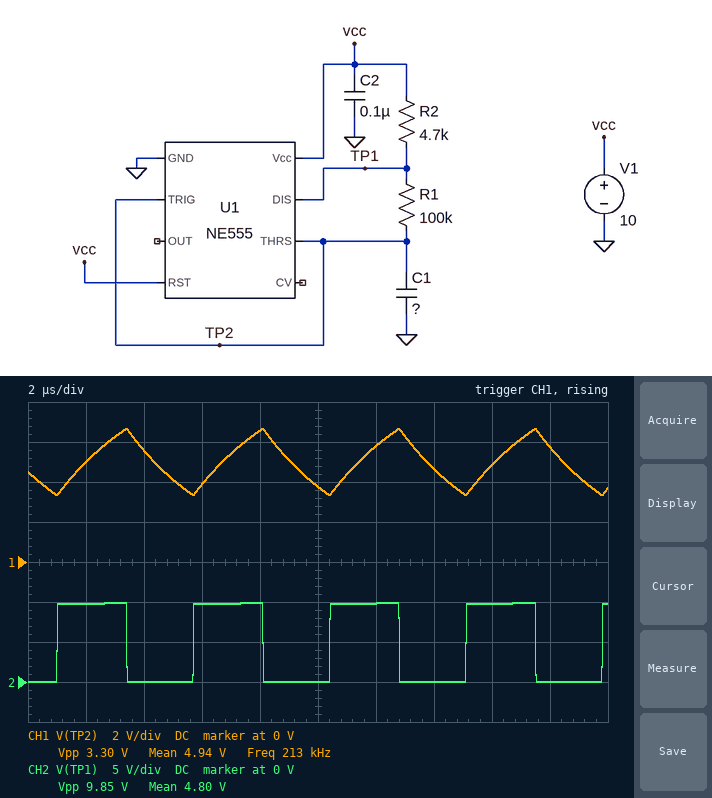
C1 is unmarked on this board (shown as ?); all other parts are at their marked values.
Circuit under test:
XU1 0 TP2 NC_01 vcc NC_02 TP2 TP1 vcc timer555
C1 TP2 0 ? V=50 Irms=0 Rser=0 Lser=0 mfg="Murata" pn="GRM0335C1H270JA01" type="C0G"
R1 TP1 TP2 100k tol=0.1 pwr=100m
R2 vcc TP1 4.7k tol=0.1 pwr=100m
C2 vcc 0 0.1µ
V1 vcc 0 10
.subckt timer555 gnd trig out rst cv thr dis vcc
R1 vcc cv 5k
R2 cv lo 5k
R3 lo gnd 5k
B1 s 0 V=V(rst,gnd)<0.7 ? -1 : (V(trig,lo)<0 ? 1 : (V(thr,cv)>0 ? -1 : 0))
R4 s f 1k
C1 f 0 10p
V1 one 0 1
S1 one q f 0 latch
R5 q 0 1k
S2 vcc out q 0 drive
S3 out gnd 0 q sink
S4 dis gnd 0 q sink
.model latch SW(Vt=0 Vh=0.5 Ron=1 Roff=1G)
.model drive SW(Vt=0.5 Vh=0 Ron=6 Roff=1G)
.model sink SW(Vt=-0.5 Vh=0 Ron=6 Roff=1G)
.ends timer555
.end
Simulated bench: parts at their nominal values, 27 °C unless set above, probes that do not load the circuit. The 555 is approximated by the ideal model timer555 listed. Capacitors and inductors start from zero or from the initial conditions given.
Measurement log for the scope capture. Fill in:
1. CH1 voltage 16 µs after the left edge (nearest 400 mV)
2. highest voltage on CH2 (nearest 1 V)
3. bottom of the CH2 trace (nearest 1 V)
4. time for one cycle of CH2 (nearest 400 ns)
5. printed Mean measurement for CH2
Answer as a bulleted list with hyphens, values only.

- 4.8 V
- 10 V
- 0 V
- 4.8 µs
- 4.80 V
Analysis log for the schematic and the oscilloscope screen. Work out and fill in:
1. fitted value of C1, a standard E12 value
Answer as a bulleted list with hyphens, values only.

- 33 pF
